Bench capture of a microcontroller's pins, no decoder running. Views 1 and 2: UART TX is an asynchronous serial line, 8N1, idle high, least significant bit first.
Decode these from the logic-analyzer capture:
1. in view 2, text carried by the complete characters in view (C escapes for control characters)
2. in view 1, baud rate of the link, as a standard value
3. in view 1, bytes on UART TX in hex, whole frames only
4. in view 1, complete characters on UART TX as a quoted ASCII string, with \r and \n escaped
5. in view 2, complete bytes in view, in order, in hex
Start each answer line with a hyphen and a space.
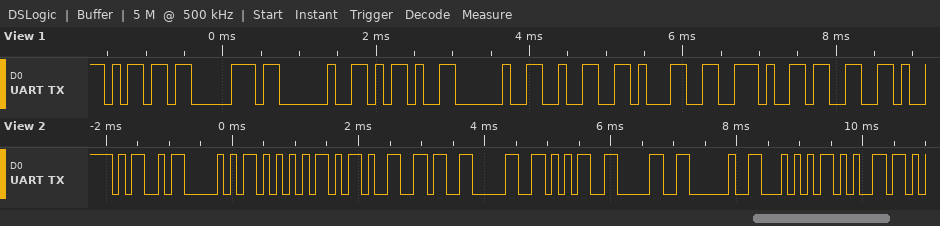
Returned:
- "MPU-6050 Te"
- 9600 baud
- 0x6D 0x70 0x20 0x2D 0x20 0x32 0x31 0x2E 0x33
- "mp - 21.3"
- 4D 50 55 2D 36 30 35 30 20 54 65
